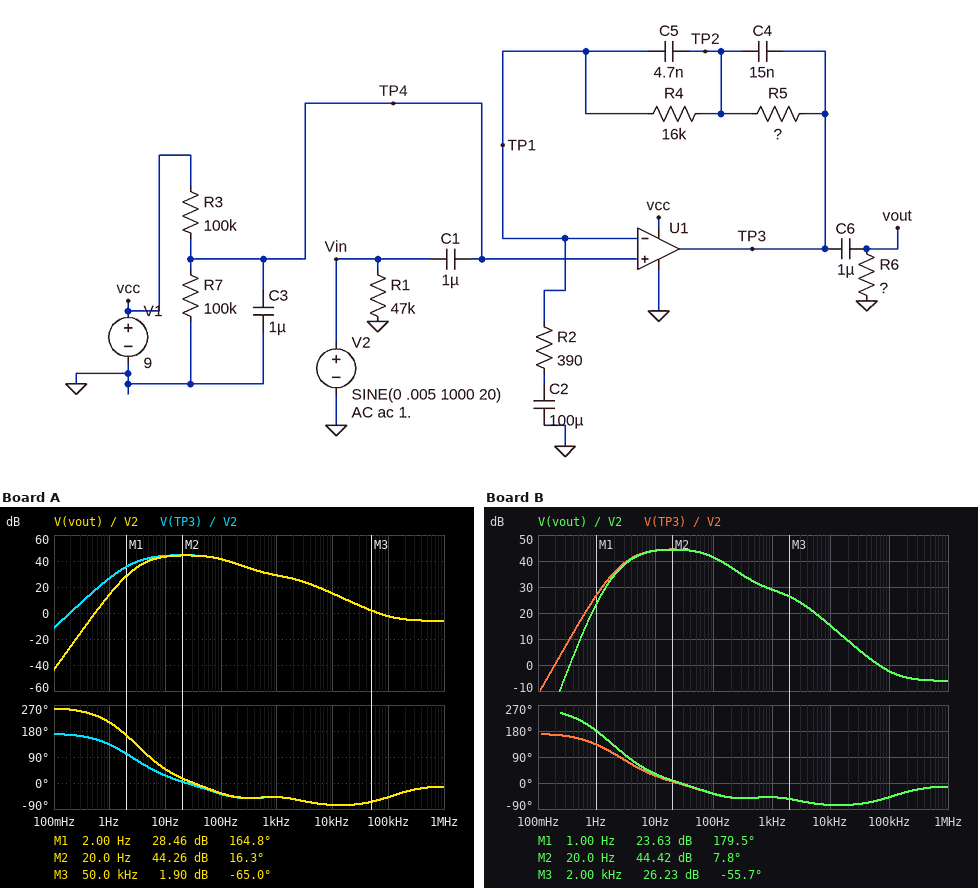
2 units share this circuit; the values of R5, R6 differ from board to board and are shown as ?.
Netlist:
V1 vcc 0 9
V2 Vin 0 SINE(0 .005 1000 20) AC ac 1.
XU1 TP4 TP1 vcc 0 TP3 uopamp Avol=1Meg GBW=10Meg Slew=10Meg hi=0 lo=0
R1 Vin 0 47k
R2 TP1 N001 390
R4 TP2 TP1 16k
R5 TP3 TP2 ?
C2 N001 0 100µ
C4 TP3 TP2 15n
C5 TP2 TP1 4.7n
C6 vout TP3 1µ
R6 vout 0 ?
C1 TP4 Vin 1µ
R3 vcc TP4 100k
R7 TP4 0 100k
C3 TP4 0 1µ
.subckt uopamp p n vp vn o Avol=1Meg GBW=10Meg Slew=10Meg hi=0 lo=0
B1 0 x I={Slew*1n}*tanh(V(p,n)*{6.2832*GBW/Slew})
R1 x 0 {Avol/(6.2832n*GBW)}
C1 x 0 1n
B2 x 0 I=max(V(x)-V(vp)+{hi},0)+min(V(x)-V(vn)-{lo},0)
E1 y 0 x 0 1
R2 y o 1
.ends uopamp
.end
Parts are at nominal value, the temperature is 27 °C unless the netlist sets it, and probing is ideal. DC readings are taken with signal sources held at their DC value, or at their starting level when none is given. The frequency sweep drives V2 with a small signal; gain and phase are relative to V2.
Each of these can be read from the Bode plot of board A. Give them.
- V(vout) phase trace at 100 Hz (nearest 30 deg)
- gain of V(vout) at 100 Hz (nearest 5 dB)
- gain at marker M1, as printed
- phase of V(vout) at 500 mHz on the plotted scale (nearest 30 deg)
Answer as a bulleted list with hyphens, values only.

- -30 deg
- 40 dB
- 28.46 dB
- 240 deg
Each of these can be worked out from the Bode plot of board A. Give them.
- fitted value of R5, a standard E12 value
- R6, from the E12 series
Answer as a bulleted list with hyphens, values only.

- 120 kΩ
- 39 kΩ
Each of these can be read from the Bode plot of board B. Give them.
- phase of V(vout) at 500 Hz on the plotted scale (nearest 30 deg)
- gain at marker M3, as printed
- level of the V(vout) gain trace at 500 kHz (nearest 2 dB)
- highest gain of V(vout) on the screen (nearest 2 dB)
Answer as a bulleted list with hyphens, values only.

- -60 deg
- 26.23 dB
- -6 dB
- 44 dB
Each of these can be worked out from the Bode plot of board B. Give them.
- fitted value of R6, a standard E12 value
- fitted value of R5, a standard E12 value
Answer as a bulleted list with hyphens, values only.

- 150 kΩ
- 120 kΩ
